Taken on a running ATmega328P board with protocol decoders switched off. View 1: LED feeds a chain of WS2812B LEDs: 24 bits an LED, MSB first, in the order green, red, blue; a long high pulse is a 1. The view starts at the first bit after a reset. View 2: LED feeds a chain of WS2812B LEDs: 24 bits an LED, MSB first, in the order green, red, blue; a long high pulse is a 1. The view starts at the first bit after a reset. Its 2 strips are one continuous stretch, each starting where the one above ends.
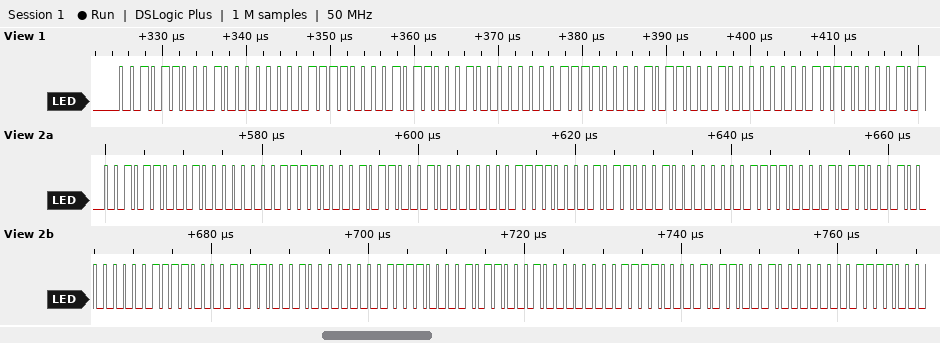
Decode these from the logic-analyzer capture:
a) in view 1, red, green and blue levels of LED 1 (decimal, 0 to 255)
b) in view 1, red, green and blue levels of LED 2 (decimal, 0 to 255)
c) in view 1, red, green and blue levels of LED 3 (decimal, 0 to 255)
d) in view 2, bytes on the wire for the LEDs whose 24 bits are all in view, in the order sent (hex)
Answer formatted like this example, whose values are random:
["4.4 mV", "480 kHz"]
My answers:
["64, 44, 60", "64, 44, 60", "64, 44, 60", "2C 40 3C 2C 40 3C 2C 40 3C 2C 40 3C 2C 40 3C 2C 40 3C 2C 40 3C"]
